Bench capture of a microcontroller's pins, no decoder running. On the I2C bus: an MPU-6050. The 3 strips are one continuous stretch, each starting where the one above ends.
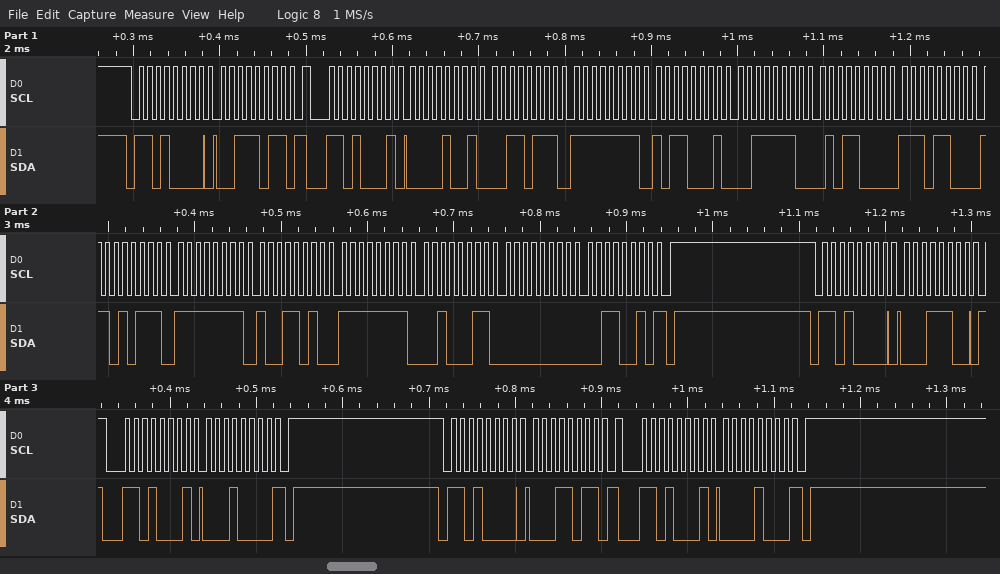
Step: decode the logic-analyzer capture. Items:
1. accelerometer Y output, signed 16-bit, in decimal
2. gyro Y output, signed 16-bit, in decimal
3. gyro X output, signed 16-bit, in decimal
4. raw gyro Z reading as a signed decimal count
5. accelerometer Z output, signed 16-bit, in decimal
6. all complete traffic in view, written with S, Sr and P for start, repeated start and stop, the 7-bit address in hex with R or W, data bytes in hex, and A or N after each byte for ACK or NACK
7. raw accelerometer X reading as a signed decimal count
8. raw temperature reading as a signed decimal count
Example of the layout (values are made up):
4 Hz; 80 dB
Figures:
-79; -221; -102; 50; 15960; S 68W A 3B A Sr 68R A 09 A 37 A FF A B1 A 3E A 58 A EC A D7 A FF A 9A A FF A 23 A 00 A 32 N P S 68W A 1C A Sr 68R A 10 N P S 68W A 1B A Sr 68R A 08 N P; 2359; -4905
